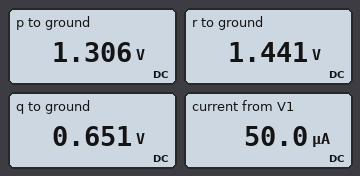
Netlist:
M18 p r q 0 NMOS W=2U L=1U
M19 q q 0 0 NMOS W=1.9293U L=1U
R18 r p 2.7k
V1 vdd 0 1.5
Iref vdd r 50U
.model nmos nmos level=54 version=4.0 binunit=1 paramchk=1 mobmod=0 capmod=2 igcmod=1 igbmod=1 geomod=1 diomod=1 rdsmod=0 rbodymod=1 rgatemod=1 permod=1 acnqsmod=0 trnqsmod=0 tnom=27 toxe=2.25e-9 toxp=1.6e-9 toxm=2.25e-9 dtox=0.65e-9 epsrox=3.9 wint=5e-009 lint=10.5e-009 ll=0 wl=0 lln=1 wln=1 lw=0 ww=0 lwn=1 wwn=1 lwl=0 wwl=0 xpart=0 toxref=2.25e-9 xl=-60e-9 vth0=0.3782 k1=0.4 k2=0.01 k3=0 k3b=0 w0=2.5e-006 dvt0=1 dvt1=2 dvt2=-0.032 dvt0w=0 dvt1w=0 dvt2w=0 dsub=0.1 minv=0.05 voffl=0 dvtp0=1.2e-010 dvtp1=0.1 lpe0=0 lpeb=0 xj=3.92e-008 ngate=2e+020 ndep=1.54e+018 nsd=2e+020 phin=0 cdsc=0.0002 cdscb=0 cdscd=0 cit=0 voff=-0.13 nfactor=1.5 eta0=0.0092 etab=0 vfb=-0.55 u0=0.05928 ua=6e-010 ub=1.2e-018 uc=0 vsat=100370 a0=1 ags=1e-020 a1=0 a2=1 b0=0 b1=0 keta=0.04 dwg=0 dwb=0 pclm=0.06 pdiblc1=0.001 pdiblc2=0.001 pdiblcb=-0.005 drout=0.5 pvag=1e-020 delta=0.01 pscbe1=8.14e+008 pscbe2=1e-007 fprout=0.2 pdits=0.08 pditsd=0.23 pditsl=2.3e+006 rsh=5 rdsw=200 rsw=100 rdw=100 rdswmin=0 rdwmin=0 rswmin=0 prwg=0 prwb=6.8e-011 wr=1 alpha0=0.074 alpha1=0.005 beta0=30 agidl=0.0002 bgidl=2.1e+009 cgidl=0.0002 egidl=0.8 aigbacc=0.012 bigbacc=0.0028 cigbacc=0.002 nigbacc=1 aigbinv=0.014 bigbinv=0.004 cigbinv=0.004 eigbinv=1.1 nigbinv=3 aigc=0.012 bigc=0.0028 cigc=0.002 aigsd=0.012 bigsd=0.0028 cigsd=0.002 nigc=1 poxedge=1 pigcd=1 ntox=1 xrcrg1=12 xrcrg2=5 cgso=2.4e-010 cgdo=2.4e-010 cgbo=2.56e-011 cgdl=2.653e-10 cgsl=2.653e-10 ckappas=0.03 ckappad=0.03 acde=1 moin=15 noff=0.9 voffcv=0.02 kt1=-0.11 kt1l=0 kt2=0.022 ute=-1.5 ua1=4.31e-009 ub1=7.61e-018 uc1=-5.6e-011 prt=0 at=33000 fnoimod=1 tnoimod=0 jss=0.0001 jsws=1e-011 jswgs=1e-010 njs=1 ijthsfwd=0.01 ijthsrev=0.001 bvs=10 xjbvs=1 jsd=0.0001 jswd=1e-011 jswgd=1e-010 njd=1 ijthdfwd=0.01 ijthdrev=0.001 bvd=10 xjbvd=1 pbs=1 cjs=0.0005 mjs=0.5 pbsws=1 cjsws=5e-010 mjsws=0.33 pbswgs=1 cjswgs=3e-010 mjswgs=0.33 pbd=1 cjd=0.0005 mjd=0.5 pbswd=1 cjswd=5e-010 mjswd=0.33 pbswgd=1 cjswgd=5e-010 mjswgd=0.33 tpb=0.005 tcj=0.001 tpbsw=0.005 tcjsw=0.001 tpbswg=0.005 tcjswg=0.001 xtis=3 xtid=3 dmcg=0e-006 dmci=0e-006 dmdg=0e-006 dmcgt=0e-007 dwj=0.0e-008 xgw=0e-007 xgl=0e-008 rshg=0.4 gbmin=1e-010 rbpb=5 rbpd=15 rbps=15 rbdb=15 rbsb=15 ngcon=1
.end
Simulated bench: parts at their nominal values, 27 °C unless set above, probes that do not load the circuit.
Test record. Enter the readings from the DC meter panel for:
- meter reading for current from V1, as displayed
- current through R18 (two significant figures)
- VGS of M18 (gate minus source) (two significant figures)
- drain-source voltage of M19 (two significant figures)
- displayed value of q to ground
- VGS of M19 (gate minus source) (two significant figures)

50.0 µA
50 µA
790 mV
650 mV
0.651 V
650 mV
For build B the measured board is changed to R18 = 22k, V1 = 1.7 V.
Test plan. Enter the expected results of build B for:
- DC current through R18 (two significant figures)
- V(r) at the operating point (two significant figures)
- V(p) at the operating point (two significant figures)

50 µA
1.8 V
730 mV
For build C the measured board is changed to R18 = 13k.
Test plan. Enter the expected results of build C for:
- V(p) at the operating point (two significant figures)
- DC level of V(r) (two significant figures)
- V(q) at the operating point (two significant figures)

830 mV
1.5 V
650 mV
